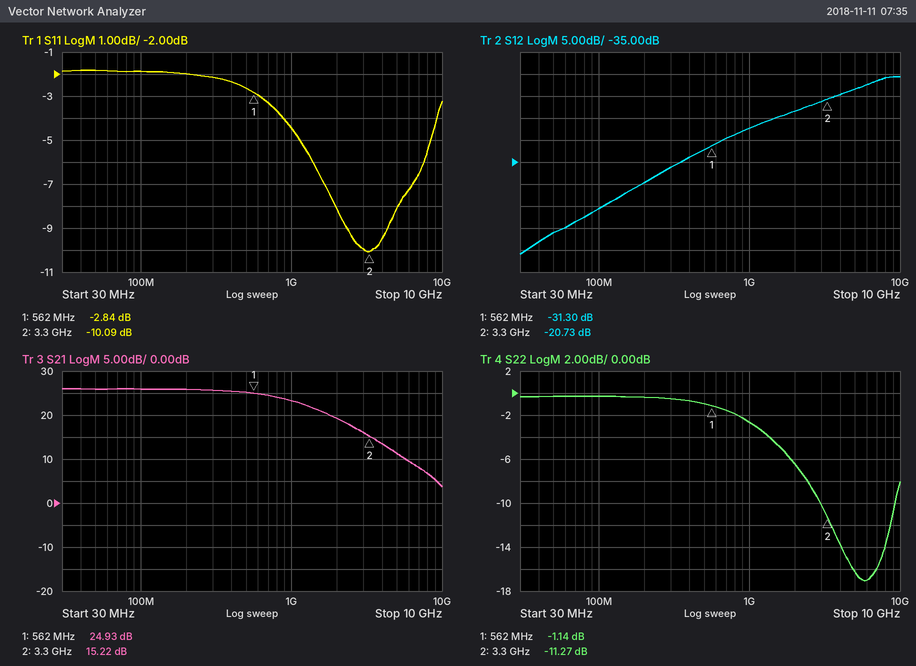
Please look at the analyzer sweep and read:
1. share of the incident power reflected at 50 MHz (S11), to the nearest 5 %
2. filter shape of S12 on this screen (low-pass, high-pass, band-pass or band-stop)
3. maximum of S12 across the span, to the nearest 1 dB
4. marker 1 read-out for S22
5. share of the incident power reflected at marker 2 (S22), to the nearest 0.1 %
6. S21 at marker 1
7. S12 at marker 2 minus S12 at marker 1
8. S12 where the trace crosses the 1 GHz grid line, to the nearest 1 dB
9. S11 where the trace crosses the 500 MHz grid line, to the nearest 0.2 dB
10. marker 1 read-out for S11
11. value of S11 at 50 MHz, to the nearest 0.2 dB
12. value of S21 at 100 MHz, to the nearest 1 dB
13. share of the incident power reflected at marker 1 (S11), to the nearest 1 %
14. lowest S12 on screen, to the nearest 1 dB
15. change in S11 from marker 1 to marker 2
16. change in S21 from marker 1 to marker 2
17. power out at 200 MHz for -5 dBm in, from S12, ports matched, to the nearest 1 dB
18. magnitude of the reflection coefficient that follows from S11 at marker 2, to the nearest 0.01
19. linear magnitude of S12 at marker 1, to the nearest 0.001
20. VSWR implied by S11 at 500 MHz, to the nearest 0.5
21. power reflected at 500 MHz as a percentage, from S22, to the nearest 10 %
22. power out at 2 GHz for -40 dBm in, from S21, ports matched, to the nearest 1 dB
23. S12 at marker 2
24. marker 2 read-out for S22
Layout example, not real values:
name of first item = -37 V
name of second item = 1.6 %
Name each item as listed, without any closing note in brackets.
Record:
share of the incident power reflected at 50 MHz (S11), to the nearest 5 % = 65 %
filter shape of S12 on this screen = high-pass
maximum of S12 across the span, to the nearest 1 dB = -16 dB
marker 1 read-out for S22 = -1.14 dB
share of the incident power reflected at marker 2 (S22), to the nearest 0.1 % = 7.5 %
S21 at marker 1 = 24.93 dB
S12 at marker 2 minus S12 at marker 1 = 10.57 dB
S12 where the trace crosses the 1 GHz grid line, to the nearest 1 dB = -27 dB
S11 where the trace crosses the 500 MHz grid line, to the nearest 0.2 dB = -2.6 dB
marker 1 read-out for S11 = -2.84 dB
value of S11 at 50 MHz, to the nearest 0.2 dB = -1.8 dB
value of S21 at 100 MHz, to the nearest 1 dB = 26 dB
share of the incident power reflected at marker 1 (S11), to the nearest 1 % = 52 %
lowest S12 on screen, to the nearest 1 dB = -56 dB
change in S11 from marker 1 to marker 2 = -7.25 dB
change in S21 from marker 1 to marker 2 = -9.71 dB
power out at 200 MHz for -5 dBm in, from S12, ports matched, to the nearest 1 dB = -45 dBm
magnitude of the reflection coefficient that follows from S11 at marker 2, to the nearest 0.01 = 0.31
linear magnitude of S12 at marker 1, to the nearest 0.001 = 0.027
VSWR implied by S11 at 500 MHz, to the nearest 0.5 = 6.5
power reflected at 500 MHz as a percentage, from S22, to the nearest 10 % = 80 %
power out at 2 GHz for -40 dBm in, from S21, ports matched, to the nearest 1 dB = -21 dBm
S12 at marker 2 = -20.73 dB
marker 2 read-out for S22 = -11.27 dB
